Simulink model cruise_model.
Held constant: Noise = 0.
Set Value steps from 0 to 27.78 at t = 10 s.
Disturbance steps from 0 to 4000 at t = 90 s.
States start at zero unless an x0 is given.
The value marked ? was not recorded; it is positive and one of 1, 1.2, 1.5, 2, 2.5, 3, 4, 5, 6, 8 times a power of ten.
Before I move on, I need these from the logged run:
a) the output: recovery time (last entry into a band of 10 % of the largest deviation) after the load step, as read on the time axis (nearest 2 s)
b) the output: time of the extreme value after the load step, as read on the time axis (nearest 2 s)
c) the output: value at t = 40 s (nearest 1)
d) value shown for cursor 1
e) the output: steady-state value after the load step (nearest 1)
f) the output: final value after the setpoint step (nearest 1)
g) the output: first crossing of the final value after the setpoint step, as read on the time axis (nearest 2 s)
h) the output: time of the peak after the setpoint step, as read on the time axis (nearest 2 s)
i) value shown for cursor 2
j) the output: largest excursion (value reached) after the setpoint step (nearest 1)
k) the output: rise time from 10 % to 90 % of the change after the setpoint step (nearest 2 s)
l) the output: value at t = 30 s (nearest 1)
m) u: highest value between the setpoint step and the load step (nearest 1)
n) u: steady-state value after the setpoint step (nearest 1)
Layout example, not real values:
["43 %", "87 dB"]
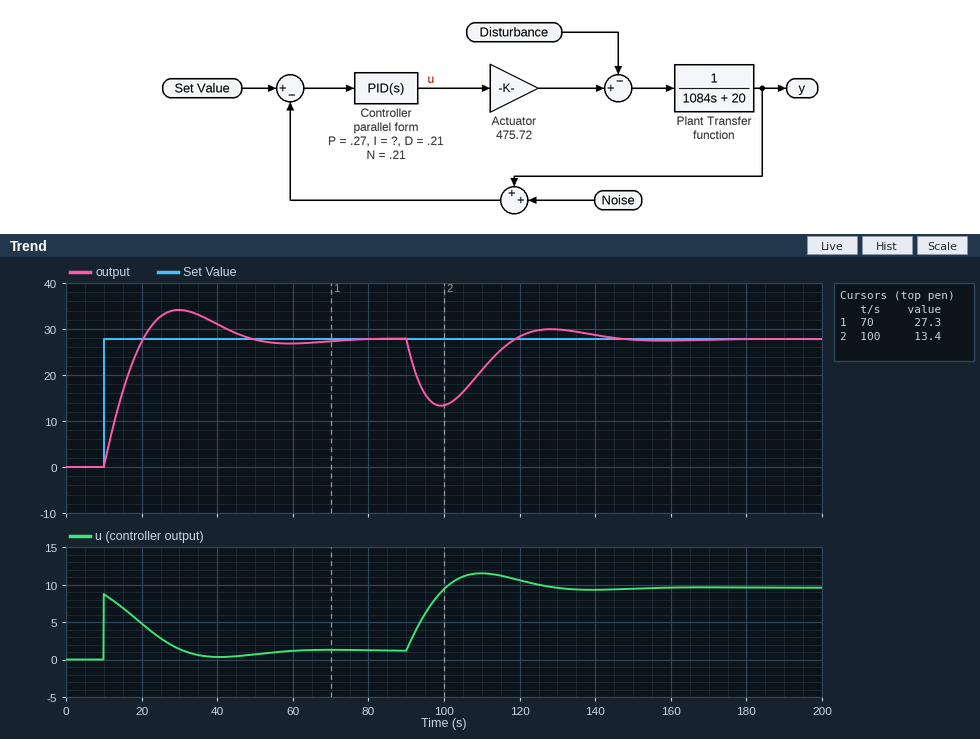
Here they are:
["136 s", "100 s", "31", "27.3", "28", "28", "20 s", "30 s", "13.4", "34", "8 s", "34", "9", "1"]
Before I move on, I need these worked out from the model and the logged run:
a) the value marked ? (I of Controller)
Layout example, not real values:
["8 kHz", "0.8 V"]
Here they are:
["0.04"]
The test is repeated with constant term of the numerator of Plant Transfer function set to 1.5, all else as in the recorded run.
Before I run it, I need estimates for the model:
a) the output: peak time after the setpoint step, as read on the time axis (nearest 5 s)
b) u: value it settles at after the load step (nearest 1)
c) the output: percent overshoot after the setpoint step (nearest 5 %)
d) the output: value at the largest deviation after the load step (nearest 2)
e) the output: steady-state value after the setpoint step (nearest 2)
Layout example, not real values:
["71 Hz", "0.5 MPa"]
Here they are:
["25 s", "9", "20 %", "12", "28"]
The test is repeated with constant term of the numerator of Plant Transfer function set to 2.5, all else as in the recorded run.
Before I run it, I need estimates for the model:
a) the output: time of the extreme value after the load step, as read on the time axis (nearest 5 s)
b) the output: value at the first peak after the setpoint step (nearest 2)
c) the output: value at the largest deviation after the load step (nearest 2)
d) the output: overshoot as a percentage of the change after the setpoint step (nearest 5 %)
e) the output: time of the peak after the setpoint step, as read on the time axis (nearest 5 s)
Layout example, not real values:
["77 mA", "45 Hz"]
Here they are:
["95 s", "32", "10", "15 %", "20 s"]
